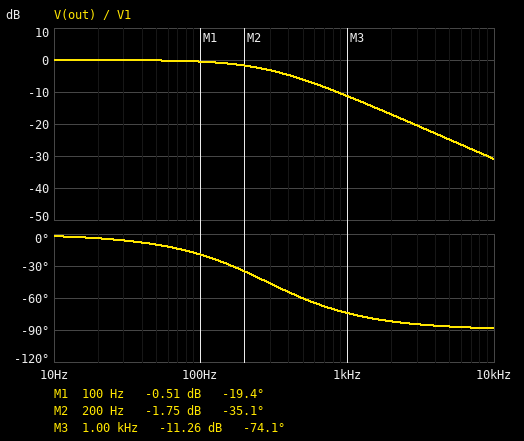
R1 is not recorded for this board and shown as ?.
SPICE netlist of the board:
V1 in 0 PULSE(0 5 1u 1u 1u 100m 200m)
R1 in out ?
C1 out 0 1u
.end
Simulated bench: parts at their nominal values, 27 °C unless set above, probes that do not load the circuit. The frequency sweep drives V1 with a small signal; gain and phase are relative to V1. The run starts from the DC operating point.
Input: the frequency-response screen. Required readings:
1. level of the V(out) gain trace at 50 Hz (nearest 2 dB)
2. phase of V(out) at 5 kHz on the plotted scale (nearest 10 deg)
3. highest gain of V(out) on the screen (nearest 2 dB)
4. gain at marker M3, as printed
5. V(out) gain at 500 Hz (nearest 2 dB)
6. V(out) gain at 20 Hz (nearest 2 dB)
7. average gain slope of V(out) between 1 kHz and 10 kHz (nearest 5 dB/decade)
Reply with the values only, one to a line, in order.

0 dB
-90 deg
0 dB
-11.26 dB
-6 dB
0 dB
-20 dB/decade
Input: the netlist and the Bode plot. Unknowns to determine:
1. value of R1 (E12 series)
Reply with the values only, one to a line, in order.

560 Ω
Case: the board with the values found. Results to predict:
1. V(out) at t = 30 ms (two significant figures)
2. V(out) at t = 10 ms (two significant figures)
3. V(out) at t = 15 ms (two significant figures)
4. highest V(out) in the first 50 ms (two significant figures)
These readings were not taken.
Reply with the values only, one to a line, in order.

5.0 V
5.0 V
5.0 V
5.0 V
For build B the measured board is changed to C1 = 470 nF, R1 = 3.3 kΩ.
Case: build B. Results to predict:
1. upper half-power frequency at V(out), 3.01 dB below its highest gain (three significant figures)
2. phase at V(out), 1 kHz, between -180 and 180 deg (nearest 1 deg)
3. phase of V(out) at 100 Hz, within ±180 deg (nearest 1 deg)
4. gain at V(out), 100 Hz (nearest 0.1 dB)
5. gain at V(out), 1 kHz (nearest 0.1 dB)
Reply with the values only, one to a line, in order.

103 Hz
-84 deg
-44 deg
-2.9 dB
-19.8 dB
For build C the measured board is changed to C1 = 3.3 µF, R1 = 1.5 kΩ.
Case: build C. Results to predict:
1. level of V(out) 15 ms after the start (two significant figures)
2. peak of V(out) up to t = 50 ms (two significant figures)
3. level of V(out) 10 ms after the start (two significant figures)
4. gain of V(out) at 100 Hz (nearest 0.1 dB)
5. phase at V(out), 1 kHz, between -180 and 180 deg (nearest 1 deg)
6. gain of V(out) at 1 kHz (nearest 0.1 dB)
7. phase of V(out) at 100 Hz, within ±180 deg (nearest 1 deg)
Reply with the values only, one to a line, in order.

4.8 V
5.0 V
4.3 V
-10.3 dB
-88 deg
-29.9 dB
-72 deg
